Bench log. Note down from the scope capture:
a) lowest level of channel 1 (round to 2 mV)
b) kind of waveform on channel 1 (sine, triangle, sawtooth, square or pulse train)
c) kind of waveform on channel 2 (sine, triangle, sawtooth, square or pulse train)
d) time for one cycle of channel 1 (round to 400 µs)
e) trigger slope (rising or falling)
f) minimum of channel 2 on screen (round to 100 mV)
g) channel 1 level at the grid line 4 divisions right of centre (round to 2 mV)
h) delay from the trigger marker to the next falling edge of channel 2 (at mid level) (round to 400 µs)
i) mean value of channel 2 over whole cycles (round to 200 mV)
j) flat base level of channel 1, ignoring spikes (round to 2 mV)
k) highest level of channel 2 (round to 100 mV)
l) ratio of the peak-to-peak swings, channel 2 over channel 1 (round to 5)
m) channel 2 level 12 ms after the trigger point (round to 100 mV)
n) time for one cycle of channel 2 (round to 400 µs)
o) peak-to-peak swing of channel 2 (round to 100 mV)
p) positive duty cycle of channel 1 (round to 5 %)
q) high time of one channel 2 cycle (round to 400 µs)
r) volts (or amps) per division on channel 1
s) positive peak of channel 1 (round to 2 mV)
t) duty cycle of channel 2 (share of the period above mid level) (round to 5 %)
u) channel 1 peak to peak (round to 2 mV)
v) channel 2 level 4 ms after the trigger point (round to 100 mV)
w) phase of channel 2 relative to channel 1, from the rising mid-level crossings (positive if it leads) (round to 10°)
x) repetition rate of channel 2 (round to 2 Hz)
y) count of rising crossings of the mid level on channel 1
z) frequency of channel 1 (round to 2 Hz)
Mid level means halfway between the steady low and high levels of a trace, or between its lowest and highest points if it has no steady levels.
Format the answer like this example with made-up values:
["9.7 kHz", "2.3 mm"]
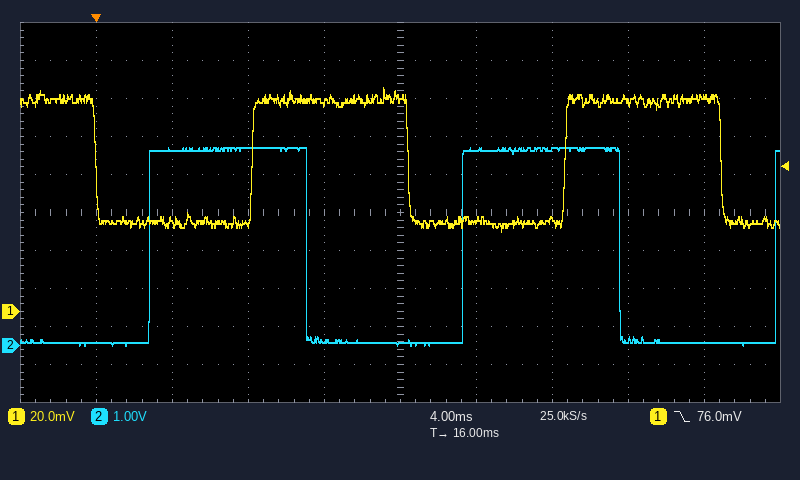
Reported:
["42 mV", "square", "square", "16.4 ms", "falling", "0.0 V", "112 mV", "11.2 ms", "2.6 V", "46 mV", "5.2 V", "70", "100 mV", "16.4 ms", "5.2 V", "50 %", "8.4 ms", "20 mV", "118 mV", "50 %", "76 mV", "5.2 V", "+120°", "60 Hz", "2", "60 Hz"]
